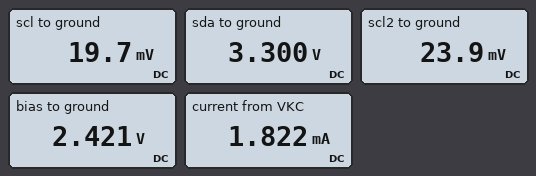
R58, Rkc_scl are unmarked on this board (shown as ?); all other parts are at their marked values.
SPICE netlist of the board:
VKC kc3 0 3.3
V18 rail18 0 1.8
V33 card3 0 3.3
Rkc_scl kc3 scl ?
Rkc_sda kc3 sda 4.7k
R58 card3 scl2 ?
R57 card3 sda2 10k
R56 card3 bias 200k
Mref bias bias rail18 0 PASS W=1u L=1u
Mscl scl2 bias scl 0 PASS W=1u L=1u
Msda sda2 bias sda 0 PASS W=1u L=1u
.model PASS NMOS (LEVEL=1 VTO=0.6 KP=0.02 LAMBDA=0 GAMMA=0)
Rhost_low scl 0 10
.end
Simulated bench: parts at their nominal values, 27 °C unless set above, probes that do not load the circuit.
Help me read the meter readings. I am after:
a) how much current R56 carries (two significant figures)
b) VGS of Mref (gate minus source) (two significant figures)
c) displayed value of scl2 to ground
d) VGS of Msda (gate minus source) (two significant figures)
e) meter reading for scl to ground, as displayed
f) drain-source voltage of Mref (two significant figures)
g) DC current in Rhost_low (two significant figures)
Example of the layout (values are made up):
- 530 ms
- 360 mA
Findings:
- 4.4 µA
- 620 mV
- 23.9 mV
- -880 mV
- 19.7 mV
- 620 mV
- 2.0 mA
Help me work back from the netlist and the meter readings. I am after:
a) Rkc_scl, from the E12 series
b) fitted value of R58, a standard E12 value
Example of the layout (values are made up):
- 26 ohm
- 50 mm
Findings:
- 1.8 kΩ
- 22 kΩ
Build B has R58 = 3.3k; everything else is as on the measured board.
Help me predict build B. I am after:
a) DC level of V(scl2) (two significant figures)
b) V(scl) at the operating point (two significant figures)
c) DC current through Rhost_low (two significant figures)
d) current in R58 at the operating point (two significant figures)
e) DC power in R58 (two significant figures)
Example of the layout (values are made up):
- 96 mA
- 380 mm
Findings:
- 56 mV
- 28 mV
- 2.8 mA
- 980 µA
- 3.2 mW
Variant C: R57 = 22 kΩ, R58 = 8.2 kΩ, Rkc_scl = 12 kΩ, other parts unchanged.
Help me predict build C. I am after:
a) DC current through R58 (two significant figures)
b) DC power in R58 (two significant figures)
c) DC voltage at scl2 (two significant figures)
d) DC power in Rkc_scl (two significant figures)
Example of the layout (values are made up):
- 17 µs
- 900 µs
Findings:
- 400 µA
- 1.3 mW
- 18 mV
- 900 µW
